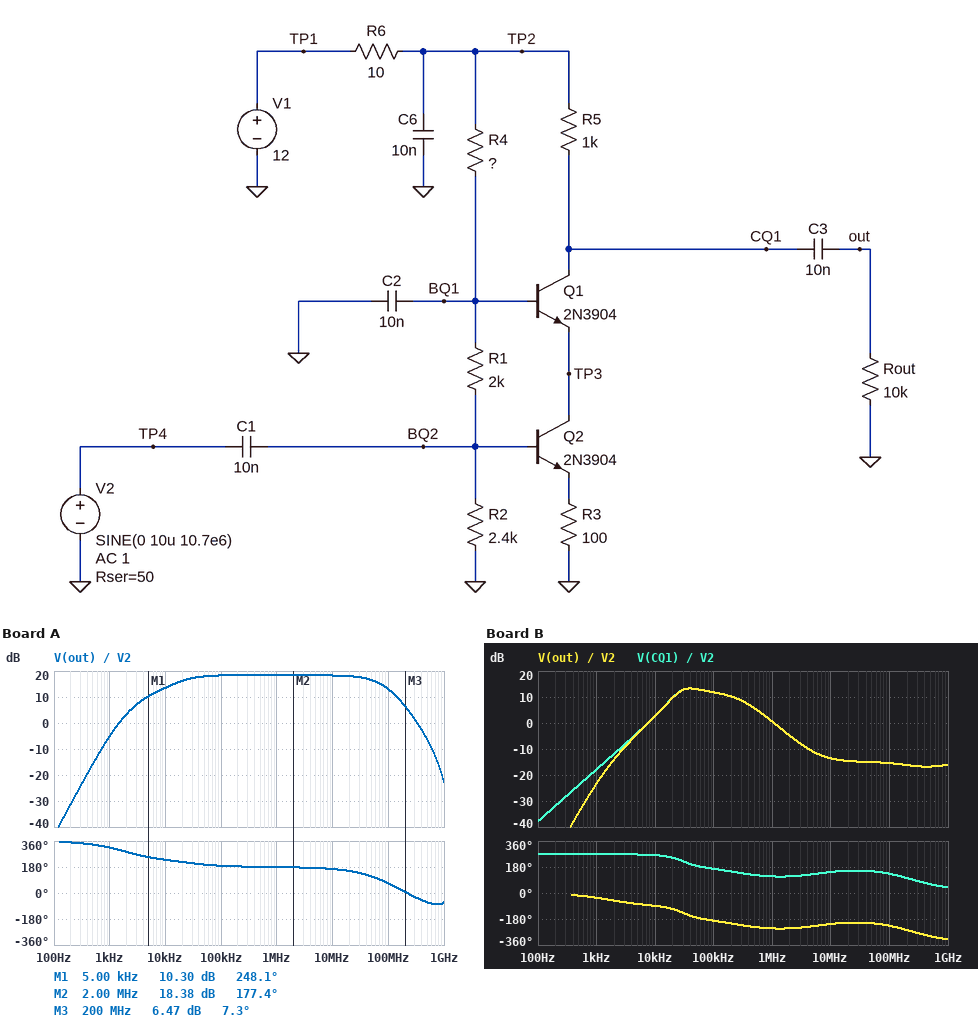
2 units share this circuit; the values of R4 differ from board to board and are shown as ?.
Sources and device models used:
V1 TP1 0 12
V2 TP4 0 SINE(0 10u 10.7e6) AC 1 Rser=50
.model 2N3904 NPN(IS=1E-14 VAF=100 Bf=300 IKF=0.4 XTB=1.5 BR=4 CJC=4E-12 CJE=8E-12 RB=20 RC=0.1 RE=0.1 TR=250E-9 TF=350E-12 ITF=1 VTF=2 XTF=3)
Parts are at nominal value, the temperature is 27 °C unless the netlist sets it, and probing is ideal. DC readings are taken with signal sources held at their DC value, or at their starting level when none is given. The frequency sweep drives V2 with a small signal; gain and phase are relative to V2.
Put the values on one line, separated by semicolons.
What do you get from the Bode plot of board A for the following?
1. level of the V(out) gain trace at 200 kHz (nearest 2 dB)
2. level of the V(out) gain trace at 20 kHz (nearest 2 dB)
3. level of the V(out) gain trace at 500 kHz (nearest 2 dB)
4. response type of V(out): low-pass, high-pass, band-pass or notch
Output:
18 dB; 16 dB; 18 dB; band-pass
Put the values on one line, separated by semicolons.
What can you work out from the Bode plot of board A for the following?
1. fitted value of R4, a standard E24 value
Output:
15 kΩ
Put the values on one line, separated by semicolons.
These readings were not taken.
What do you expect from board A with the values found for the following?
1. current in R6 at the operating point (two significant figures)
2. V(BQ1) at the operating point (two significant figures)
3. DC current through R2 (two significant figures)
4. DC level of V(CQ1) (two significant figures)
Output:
7.4 mA; 2.6 V; 580 µA; 5.2 V
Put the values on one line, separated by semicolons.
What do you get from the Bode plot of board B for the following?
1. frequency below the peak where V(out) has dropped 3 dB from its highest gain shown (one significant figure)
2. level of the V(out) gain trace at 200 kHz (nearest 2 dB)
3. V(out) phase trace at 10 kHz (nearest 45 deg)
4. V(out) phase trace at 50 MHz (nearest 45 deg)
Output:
20 kHz; 10 dB; -90 deg; -225 deg
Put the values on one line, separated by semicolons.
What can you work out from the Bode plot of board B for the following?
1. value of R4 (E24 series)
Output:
11 kΩ
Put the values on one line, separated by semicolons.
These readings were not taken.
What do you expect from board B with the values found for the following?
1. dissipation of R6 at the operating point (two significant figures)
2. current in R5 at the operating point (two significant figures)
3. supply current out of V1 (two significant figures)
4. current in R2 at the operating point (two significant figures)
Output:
1.0 mW; 9.4 mA; 10 mA; 690 µA
